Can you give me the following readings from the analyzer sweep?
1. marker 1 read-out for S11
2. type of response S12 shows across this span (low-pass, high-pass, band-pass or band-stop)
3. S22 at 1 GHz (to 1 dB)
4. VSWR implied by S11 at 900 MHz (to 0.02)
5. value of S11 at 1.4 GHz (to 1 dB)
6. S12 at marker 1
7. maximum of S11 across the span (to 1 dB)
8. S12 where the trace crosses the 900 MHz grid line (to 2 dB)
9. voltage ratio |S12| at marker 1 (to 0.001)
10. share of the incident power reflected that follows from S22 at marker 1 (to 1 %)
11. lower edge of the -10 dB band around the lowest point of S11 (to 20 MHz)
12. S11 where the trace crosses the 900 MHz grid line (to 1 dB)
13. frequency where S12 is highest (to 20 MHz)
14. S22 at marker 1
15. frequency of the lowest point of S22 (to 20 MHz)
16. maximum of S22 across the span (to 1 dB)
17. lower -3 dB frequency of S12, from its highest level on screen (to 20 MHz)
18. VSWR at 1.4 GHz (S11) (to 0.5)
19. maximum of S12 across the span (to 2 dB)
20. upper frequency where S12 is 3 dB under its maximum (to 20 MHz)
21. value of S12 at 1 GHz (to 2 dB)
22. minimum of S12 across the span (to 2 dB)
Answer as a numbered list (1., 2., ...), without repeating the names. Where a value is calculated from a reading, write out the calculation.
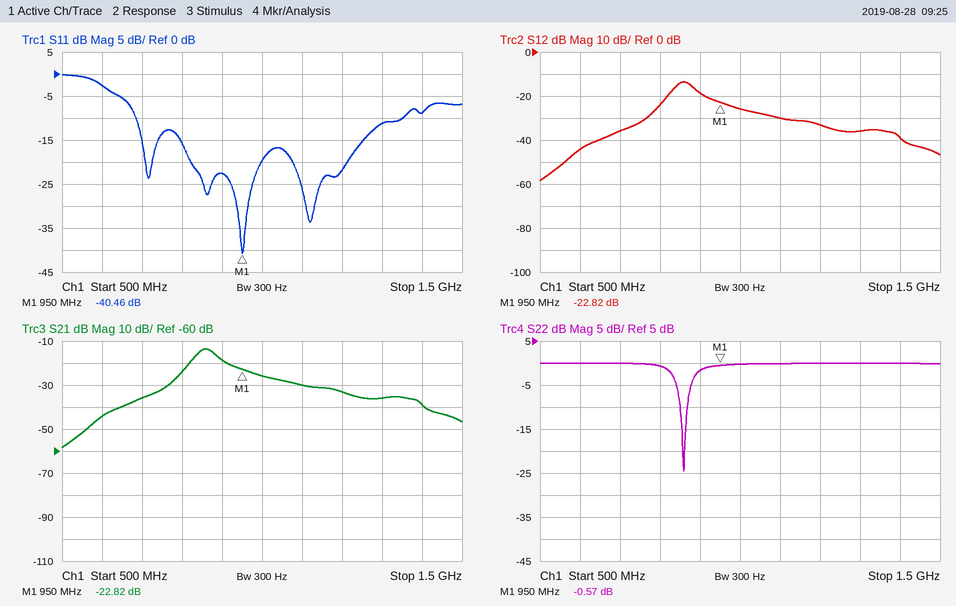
1. -40.46 dB
2. band-pass
3. 0 dB
4. |Γ| = 10^(-23/20) = 0.0708; VSWR = (1 + 0.0708)/(1 − 0.0708) ≈ 1.15, so 1.16 to the nearest 0.02
5. -9 dB
6. -22.82 dB
7. 0 dB
8. -18 dB
9. 10^(-22.82/20) ≈ 0.072
10. 10^(-0.57/10) ≈ 88 %
11. 680 MHz
12. -23 dB
13. 860 MHz
14. -0.57 dB
15. 860 MHz
16. 0 dB
17. 840 MHz
18. |Γ| = 10^(-9/20) = 0.3548; VSWR = (1 + 0.3548)/(1 − 0.3548) ≈ 2.10, so 2.0 to the nearest 0.5
19. -14 dB
20. 880 MHz
21. -26 dB
22. -58 dB
